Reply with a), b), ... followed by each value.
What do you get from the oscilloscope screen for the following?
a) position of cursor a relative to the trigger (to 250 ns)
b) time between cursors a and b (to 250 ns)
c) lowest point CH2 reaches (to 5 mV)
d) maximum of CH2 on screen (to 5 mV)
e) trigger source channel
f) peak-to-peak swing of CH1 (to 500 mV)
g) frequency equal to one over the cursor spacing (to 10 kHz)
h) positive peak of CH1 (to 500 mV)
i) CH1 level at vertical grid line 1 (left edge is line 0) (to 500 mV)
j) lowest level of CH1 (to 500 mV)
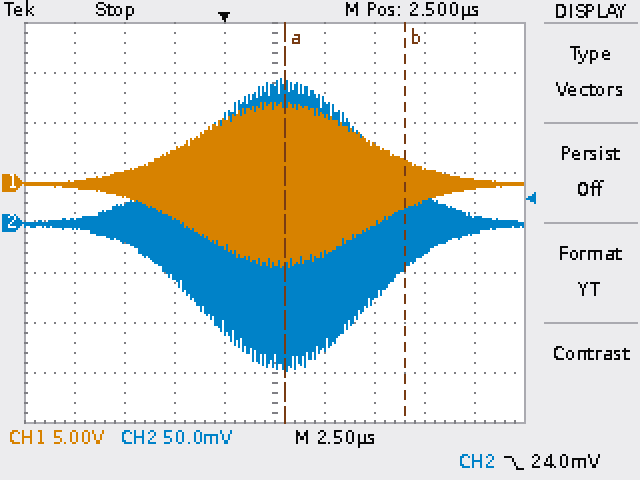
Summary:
a) +3.00 µs
b) 6.00 µs
c) -150 mV
d) 145 mV
e) CH2
f) 16.5 V
g) 170 kHz
h) 8.0 V
i) 0.0 V
j) -8.5 V
